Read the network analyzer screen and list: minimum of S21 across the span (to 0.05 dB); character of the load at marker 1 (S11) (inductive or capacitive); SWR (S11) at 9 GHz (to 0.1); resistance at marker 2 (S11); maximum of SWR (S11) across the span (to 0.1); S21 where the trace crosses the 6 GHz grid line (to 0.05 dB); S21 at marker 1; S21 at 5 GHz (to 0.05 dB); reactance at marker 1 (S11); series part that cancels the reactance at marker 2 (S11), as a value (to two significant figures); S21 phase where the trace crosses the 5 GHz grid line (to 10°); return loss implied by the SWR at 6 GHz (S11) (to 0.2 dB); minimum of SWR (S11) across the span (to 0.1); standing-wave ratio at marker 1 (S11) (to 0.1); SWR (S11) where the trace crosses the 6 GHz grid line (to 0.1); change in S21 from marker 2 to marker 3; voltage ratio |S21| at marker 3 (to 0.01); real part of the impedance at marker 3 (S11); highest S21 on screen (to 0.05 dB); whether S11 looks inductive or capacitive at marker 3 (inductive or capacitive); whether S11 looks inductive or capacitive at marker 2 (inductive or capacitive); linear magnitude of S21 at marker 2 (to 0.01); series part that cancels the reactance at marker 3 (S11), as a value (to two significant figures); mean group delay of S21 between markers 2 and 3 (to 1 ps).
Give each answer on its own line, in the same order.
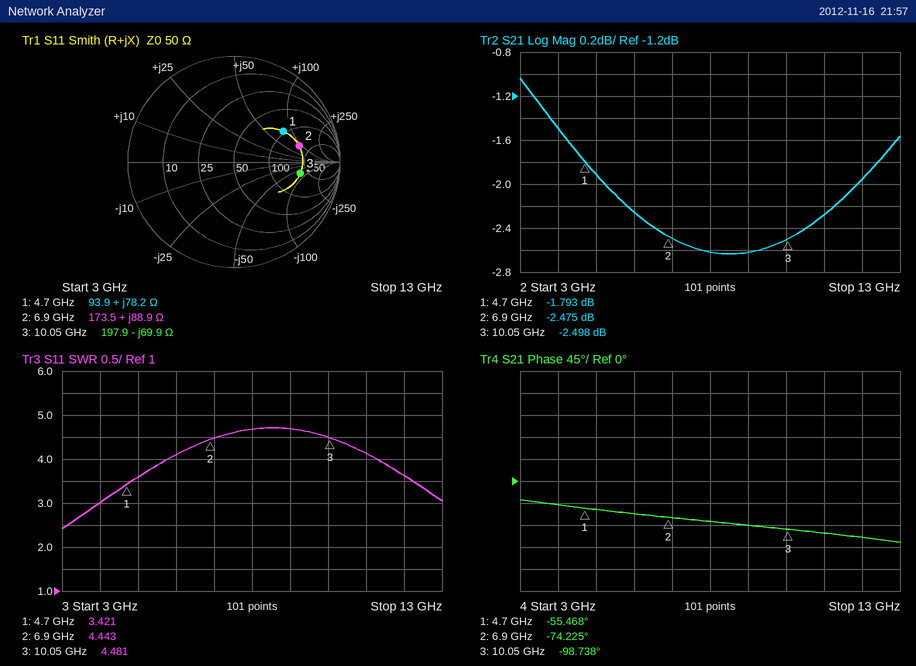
-2.65 dB
inductive
4.7
173.5 Ω
4.7
-2.25 dB
-1.793 dB
-1.90 dB
+78.2 Ω
260 fF
-60°
4.4 dB
2.4
3.4
4.1
-0.023 dB
0.75
197.9 Ω
-1.05 dB
capacitive
inductive
0.75
1.1 nH
22 ps
